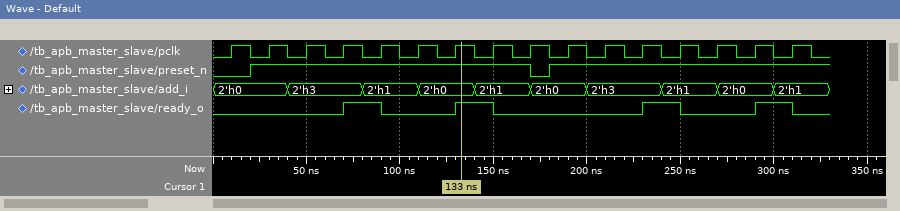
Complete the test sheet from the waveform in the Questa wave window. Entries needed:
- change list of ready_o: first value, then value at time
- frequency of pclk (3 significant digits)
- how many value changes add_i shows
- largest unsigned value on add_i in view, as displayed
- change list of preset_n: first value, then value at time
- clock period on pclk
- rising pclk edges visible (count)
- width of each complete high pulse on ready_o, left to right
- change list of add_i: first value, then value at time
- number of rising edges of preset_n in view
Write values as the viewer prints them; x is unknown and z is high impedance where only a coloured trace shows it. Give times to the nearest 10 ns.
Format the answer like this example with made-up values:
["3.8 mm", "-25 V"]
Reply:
["0, 1 at 70 ns, 0 at 90 ns, 1 at 130 ns, 0 at 150 ns, 1 at 230 ns, 0 at 250 ns, 1 at 290 ns, 0 at 310 ns", "50.0 MHz", "9", "2'h3", "0, 1 at 20 ns, 0 at 170 ns, 1 at 180 ns", "20 ns", "16", "20 ns, 20 ns, 20 ns, 20 ns", "2'h0, 2'h3 at 40 ns, 2'h1 at 80 ns, 2'h0 at 110 ns, 2'h1 at 140 ns, 2'h0 at 170 ns, 2'h3 at 200 ns, 2'h1 at 240 ns, 2'h0 at 270 ns, 2'h1 at 300 ns", "2"]
